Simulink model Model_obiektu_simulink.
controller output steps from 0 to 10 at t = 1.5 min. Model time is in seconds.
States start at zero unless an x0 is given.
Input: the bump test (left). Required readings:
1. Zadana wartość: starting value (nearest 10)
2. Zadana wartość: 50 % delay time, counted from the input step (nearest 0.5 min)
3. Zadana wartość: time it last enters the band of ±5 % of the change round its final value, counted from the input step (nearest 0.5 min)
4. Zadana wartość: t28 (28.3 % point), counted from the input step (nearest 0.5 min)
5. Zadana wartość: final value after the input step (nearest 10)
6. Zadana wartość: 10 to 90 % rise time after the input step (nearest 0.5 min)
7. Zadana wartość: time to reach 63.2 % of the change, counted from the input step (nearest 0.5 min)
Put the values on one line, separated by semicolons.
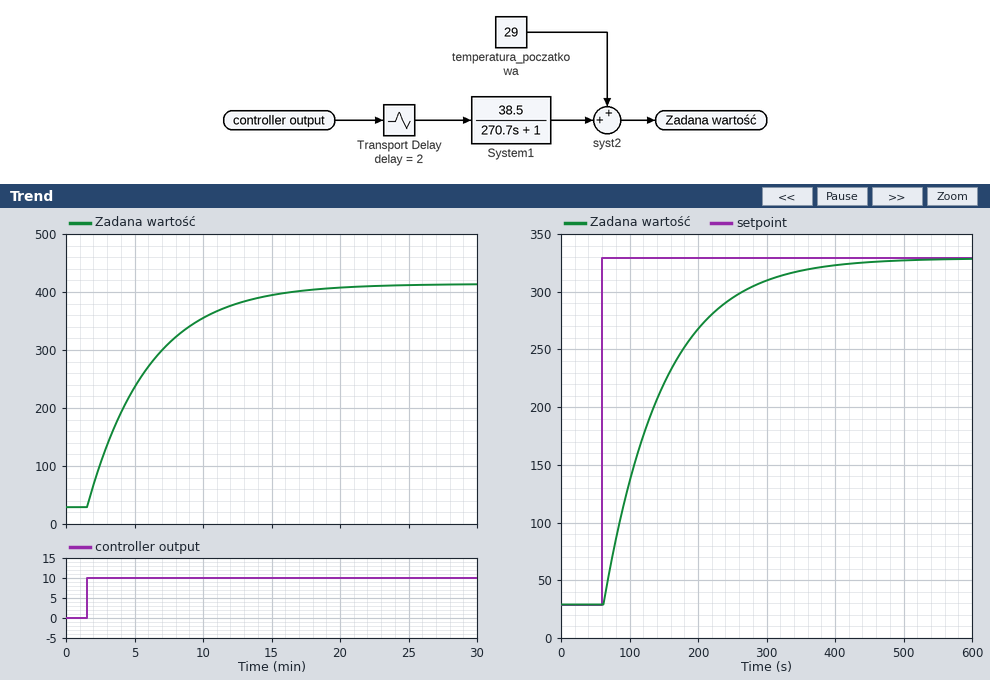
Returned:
30; 3.0 min; 13.5 min; 1.5 min; 410; 10.0 min; 4.5 min
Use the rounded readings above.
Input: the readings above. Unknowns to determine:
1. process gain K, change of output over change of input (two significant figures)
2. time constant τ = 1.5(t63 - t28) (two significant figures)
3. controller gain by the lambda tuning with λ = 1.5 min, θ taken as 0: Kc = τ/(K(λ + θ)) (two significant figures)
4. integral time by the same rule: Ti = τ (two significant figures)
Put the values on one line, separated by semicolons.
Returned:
38; 4.5 min; 0.079; 4.5 min
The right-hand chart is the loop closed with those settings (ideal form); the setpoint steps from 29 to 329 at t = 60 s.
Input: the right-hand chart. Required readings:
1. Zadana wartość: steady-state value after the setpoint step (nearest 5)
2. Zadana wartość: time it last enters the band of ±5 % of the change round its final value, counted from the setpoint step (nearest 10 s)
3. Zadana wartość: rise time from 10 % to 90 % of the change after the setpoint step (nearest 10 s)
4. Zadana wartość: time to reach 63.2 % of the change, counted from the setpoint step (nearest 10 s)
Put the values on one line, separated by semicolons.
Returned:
330; 260 s; 190 s; 90 s
